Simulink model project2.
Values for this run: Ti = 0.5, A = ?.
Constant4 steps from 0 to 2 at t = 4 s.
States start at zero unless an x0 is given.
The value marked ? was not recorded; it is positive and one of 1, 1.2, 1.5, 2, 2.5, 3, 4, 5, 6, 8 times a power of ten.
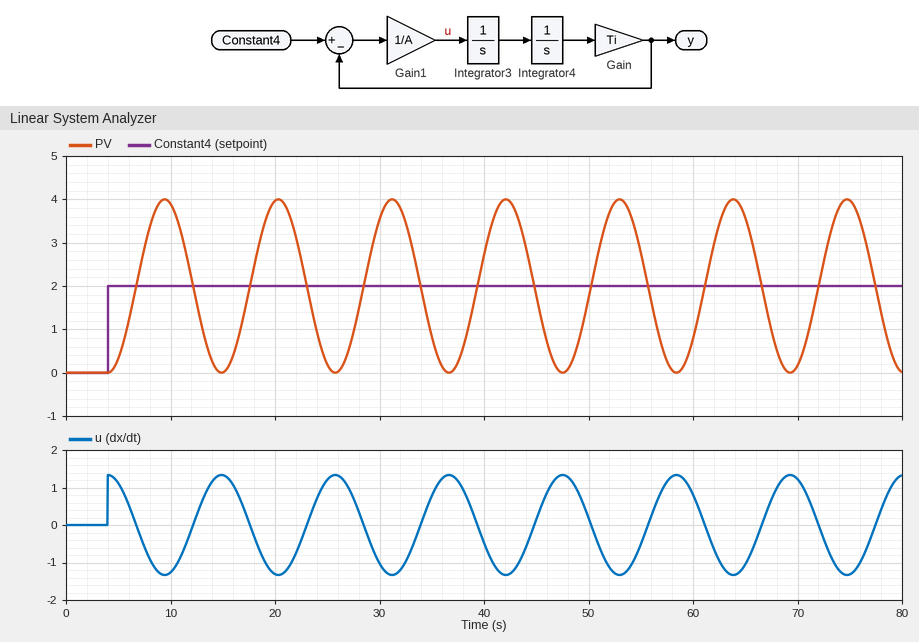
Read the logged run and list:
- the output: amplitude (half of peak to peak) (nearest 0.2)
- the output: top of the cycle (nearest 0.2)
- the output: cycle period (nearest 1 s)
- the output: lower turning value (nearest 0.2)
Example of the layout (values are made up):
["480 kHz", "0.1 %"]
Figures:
["2.0", "4.0", "11 s", "0.0"]
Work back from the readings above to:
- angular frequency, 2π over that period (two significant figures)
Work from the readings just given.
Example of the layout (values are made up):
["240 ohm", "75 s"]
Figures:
["0.57 rad/s"]
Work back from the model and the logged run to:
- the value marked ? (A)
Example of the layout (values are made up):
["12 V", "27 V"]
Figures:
["1.5"]
